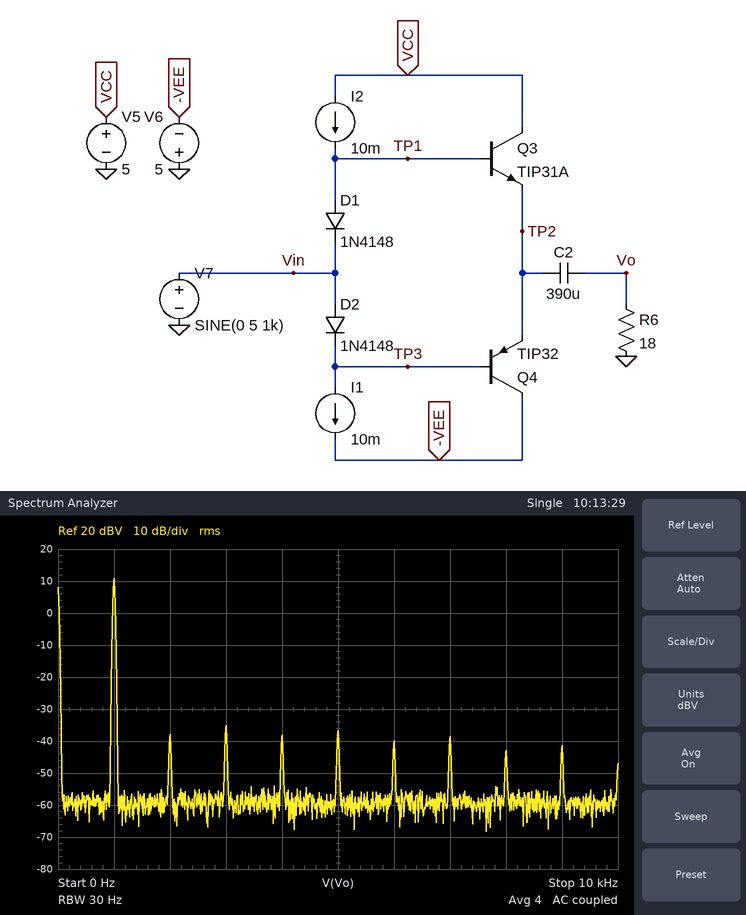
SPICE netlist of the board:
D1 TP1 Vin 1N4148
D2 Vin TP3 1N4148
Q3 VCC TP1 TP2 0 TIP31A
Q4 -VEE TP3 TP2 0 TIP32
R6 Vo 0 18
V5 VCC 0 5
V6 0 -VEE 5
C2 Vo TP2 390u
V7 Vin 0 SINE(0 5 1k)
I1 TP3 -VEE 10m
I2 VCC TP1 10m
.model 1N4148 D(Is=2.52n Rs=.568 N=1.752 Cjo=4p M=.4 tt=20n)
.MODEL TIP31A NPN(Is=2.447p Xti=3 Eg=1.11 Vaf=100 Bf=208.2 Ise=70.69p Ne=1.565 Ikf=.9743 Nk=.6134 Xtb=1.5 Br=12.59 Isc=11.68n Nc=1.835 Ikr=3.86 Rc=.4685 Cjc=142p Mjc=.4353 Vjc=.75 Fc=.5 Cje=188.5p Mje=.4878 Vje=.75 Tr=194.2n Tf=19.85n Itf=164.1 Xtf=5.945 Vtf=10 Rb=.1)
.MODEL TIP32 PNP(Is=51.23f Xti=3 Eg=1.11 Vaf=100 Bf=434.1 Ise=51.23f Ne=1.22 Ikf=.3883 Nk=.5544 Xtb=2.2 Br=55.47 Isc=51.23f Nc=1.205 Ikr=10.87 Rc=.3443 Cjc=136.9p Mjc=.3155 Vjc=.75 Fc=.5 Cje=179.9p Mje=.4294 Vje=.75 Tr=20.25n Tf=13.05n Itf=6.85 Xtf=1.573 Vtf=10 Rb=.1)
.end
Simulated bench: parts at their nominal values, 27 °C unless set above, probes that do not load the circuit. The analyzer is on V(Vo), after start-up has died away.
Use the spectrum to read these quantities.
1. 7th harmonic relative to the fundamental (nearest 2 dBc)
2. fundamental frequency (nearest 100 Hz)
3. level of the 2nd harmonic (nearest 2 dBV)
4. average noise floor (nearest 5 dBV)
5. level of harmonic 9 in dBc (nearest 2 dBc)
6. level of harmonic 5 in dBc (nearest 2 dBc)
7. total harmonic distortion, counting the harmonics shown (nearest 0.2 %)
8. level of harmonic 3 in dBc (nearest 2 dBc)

-50 dBc
1.0 kHz
-38 dBV
-60 dBV
-52 dBc
-48 dBc
1.0 %
-46 dBc
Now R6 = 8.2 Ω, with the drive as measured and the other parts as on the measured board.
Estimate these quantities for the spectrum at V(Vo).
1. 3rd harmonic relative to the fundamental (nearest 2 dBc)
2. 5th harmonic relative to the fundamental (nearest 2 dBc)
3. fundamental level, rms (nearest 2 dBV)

-36 dBc
-40 dBc
10 dBV
